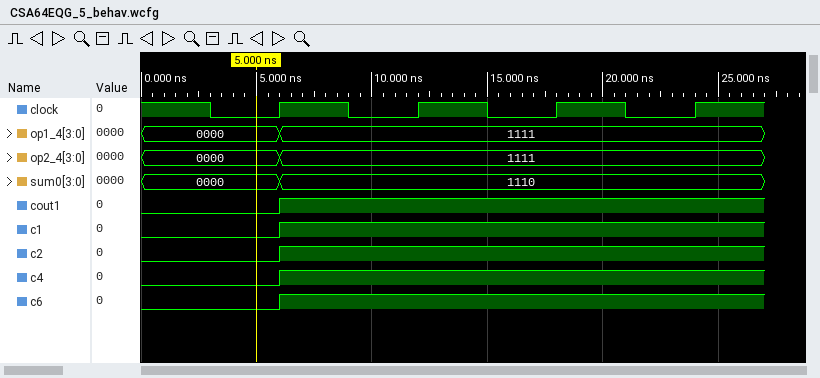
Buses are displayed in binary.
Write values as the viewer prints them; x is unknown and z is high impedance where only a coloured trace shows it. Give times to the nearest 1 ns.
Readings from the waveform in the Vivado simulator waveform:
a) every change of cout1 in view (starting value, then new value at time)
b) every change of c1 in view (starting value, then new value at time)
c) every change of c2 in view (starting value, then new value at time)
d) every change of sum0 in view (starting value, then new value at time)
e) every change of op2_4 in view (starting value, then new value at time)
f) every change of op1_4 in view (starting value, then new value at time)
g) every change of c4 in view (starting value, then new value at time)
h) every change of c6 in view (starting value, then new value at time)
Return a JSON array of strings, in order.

["0, 1 at 6 ns", "0, 1 at 6 ns", "0, 1 at 6 ns", "0000, 1110 at 6 ns", "0000, 1111 at 6 ns", "0000, 1111 at 6 ns", "0, 1 at 6 ns", "0, 1 at 6 ns"]
